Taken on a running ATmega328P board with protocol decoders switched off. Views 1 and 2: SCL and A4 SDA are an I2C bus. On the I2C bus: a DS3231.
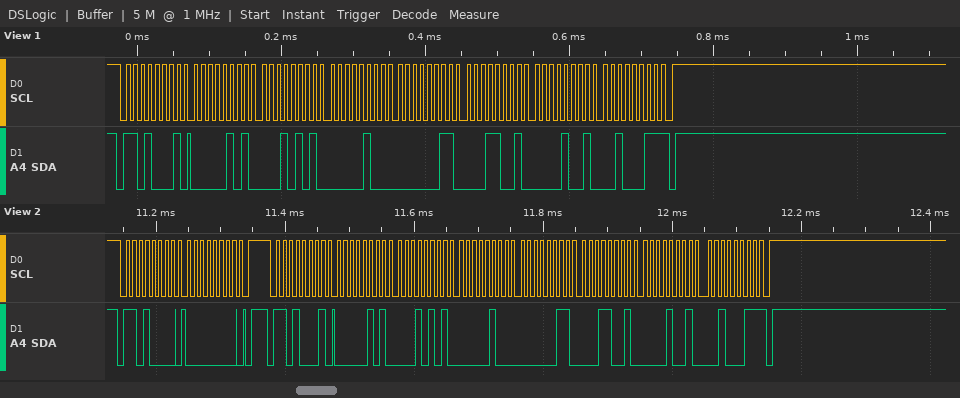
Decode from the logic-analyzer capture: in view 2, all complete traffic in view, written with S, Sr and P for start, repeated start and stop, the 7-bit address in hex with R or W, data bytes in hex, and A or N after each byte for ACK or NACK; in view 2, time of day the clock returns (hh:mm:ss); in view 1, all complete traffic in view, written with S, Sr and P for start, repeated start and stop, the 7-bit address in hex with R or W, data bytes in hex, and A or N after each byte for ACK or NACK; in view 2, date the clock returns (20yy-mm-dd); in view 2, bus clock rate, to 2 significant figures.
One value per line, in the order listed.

S 68W A 00 A P S 68R A 05 A 15 A 04 A 03 A 19 A 09 A 23 N P
04:15:05
S 68R A 05 A 15 A 04 A 03 A 19 A 09 A 23 N P
2023-09-19
100 kHz
